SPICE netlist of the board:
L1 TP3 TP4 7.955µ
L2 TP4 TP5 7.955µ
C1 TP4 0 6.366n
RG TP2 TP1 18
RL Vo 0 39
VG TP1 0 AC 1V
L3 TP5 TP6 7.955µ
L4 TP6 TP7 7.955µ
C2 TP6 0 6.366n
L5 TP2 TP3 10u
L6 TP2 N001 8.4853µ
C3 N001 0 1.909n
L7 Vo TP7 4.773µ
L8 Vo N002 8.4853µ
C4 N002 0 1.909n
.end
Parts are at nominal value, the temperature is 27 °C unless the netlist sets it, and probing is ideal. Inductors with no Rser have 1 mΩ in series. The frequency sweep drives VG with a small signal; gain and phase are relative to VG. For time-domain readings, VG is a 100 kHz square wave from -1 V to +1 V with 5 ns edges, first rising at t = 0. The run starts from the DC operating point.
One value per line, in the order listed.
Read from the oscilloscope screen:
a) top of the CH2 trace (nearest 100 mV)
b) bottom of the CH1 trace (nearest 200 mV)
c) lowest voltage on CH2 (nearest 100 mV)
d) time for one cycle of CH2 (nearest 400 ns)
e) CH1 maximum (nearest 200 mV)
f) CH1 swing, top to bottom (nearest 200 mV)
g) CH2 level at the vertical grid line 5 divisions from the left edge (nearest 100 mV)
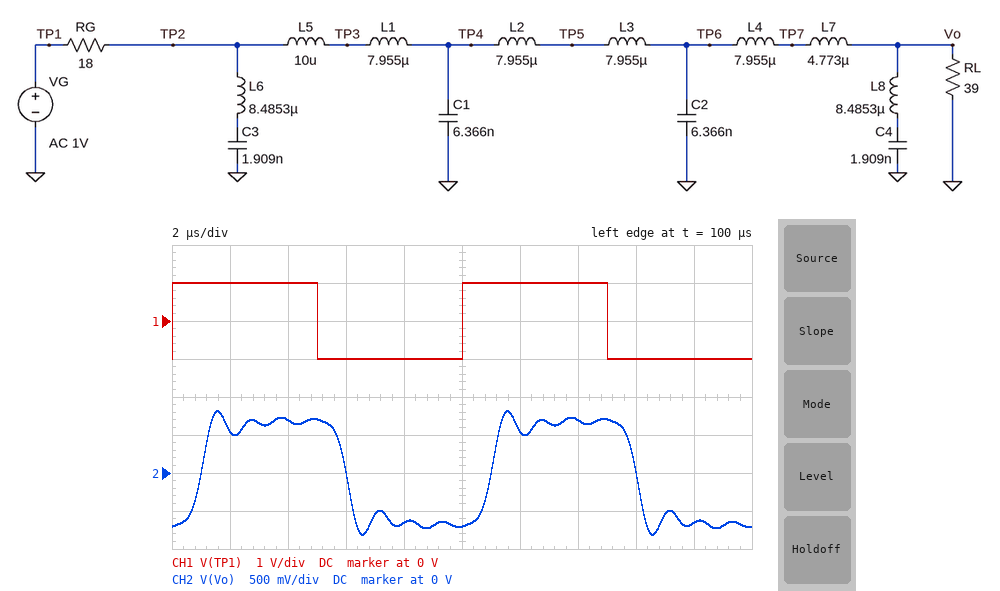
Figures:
800 mV
-1.0 V
-800 mV
10.0 µs
1.0 V
2.0 V
-700 mV
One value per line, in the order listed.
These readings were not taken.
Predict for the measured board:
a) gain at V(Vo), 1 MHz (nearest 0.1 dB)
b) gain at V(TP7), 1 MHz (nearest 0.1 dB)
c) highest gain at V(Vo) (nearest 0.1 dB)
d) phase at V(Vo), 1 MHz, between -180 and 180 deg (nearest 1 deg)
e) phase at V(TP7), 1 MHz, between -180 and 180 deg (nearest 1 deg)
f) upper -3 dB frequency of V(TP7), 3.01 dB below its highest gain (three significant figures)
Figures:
-16.9 dB
-19.2 dB
-3.3 dB
-127 deg
-37 deg
682 kHz
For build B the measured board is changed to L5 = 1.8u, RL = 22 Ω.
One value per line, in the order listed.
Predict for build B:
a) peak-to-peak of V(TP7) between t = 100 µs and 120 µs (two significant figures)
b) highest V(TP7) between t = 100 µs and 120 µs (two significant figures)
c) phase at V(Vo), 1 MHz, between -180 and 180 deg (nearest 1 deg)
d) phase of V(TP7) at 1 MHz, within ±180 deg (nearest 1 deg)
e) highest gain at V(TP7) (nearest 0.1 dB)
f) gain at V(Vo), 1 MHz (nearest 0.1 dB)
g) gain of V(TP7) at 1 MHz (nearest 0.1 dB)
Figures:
1.2 V
610 mV
-81 deg
9 deg
-3.4 dB
-10.9 dB
-8.2 dB
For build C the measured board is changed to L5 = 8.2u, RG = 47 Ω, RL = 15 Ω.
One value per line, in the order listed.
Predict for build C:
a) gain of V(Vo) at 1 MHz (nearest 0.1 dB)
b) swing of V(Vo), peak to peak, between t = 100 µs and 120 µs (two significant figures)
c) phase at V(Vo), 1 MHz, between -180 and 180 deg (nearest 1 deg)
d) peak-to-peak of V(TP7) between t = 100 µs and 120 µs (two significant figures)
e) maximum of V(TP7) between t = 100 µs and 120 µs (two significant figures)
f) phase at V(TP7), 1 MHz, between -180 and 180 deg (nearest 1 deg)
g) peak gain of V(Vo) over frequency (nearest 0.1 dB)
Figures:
-24.9 dB
680 mV
-135 deg
880 mV
440 mV
-45 deg
-11.1 dB
